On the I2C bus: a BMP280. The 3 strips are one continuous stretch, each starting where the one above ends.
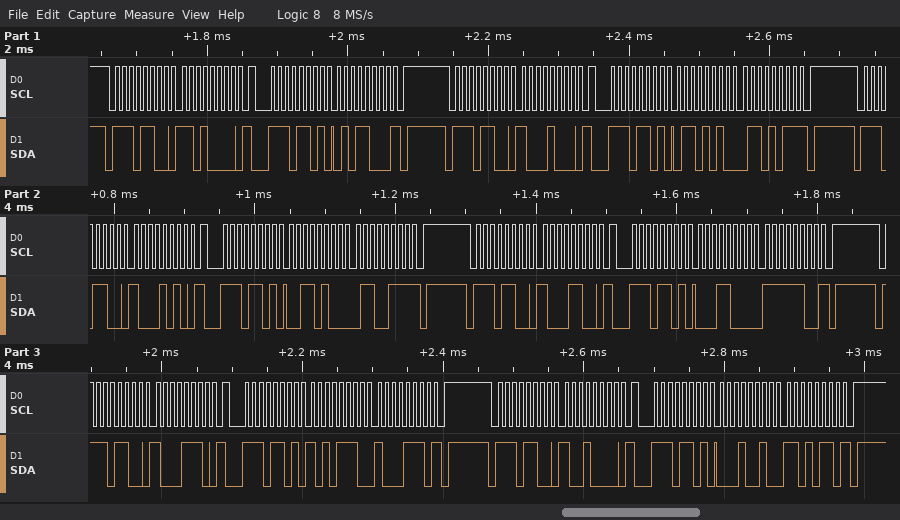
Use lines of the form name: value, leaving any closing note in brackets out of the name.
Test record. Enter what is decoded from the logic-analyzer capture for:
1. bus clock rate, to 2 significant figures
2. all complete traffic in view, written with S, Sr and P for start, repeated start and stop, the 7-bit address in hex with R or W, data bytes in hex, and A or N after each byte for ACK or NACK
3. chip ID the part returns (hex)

bus clock rate, to 2 significant figures: 100 kHz
all complete traffic in view, written with S, Sr and P for start, repeated start and stop, the 7-bit address in hex with R or W, data bytes in hex, and A or N after each byte for ACK or NACK: S 76W A D0 A Sr 76R A 58 N P S 76W A 88 A Sr 76R A 6A A 6B N P S 76W A 8A A Sr 76R A 34 A 67 N P S 76W A 8C A Sr 76R A 18 A FC N P S 76W A 8E A Sr 76R A AE A 8E N P S 76W A 90 A Sr 76R A 12 A D6 N P
chip ID the part returns: 0x58
